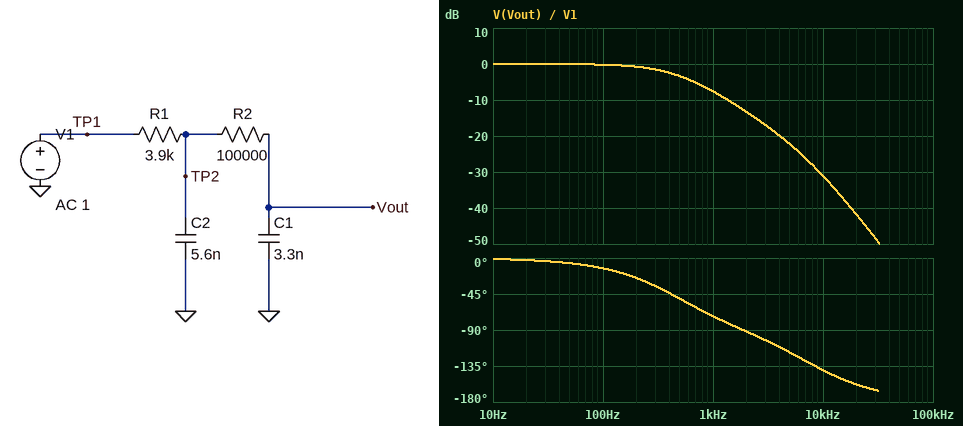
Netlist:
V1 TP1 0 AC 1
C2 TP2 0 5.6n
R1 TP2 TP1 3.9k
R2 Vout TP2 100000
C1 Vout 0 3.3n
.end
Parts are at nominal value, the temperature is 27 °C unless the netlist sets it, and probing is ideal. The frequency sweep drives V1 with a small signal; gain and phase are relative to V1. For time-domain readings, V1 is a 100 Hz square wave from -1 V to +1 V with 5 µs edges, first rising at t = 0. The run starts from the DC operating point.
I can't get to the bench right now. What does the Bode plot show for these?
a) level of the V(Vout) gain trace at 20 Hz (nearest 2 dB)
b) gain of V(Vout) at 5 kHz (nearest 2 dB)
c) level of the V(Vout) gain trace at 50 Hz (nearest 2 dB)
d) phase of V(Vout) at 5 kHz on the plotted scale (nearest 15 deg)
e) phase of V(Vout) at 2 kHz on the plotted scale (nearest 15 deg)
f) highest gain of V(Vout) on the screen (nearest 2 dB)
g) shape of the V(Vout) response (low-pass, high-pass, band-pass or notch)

0 dB
-22 dB
0 dB
-120 deg
-90 deg
0 dB
low-pass
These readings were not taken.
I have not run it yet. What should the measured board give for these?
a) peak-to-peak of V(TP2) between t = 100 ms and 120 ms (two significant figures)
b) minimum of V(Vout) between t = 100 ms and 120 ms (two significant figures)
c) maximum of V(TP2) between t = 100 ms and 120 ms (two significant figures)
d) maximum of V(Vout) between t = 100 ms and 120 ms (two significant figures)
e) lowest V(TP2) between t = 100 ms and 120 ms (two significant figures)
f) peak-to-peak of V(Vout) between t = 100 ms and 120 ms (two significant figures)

2.0 V
-1.0 V
1.0 V
1.0 V
-1.0 V
2.0 V
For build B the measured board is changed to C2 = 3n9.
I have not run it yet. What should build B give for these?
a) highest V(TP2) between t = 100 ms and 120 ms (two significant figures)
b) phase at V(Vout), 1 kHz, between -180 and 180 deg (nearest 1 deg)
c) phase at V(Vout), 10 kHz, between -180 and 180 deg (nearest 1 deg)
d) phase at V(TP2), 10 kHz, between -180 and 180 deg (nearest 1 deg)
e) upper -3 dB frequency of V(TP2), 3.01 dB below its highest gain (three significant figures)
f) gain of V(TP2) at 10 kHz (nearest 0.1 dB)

1.0 V
-70 deg
-130 deg
-43 deg
10.0 kHz
-3.0 dB
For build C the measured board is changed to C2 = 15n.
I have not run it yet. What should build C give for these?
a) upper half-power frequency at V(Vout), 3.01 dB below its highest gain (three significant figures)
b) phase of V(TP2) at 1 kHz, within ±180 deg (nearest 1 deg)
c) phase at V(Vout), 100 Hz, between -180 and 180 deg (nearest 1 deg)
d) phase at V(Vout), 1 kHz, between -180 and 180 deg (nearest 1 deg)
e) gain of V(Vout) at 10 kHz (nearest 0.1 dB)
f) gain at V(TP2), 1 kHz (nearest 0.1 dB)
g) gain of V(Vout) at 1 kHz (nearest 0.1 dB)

449 Hz
-20 deg
-14 deg
-85 deg
-38.0 dB
-0.8 dB
-8.1 dB
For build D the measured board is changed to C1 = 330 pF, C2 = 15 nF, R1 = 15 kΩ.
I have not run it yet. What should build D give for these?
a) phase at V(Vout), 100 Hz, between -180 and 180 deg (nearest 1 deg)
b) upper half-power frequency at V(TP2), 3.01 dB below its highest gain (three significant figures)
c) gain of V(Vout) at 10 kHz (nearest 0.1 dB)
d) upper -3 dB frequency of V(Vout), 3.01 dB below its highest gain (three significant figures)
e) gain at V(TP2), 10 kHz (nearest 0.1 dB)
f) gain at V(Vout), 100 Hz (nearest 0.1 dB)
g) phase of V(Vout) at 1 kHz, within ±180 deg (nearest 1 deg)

-9 deg
690 Hz
-30.3 dB
677 Hz
-23.1 dB
-0.1 dB
-67 deg
